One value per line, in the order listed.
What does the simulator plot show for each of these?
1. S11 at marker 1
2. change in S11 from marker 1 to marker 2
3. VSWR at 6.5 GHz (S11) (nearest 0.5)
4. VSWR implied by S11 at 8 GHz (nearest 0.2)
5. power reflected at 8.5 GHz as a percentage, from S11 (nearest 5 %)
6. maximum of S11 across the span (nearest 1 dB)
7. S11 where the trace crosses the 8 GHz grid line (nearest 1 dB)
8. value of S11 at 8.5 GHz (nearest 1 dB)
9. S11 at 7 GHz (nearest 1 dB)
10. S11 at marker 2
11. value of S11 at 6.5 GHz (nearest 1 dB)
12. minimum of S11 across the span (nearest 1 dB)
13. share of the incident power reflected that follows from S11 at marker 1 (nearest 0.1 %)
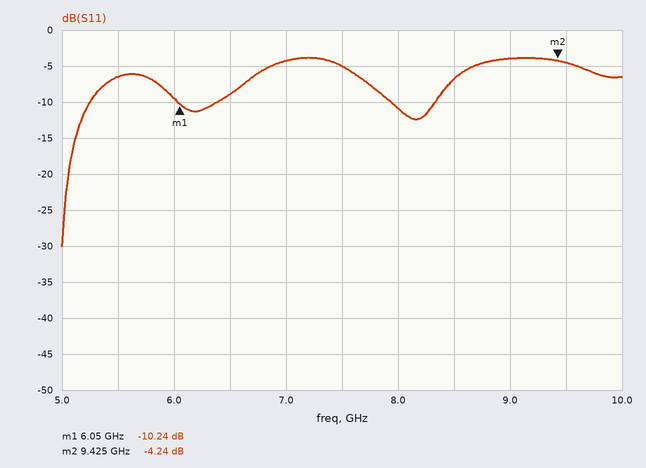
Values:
-10.24 dB
6.00 dB
2.0
1.8
20 %
-4 dB
-11 dB
-7 dB
-4 dB
-4.24 dB
-9 dB
-30 dB
9.5 %
